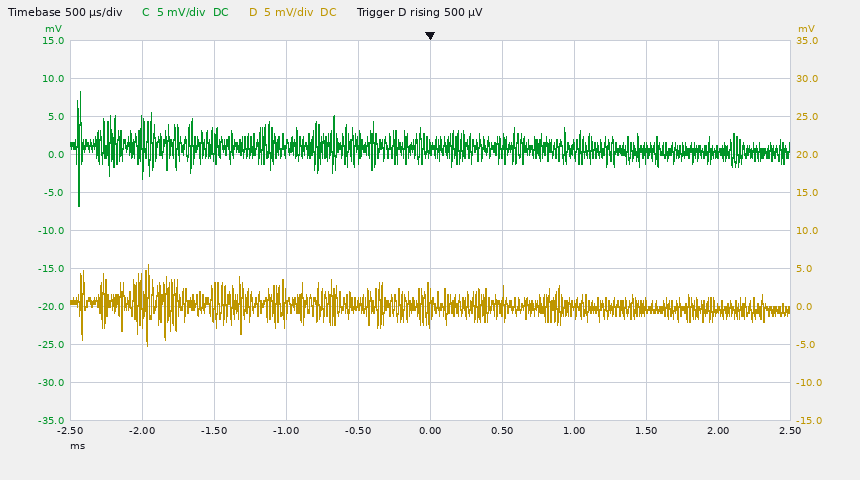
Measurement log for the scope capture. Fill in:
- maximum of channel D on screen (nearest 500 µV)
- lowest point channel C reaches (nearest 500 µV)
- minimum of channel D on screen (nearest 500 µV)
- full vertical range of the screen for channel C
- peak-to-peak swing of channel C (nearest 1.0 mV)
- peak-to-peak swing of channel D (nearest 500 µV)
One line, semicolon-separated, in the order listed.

5.5 mV; -6.5 mV; -5.0 mV; 50 mV; 15.0 mV; 10.5 mV
